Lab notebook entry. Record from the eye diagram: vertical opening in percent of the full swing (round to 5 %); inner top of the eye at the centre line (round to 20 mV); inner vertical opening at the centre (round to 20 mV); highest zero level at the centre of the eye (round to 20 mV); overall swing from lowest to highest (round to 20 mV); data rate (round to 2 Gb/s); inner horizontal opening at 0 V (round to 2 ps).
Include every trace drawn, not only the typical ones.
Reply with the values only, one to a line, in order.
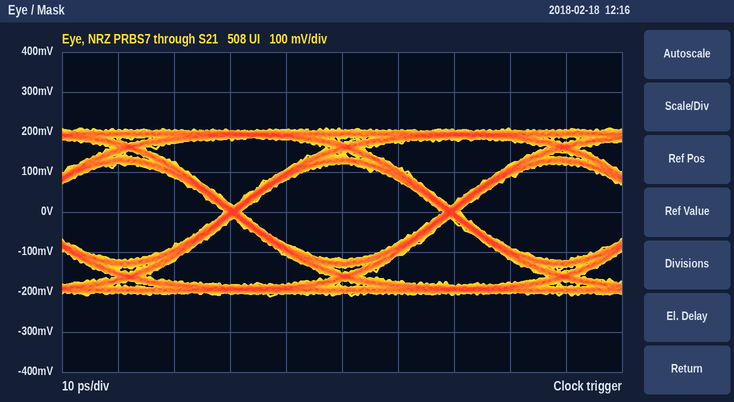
55 %
120 mV
240 mV
-120 mV
420 mV
26 Gb/s
36 ps
